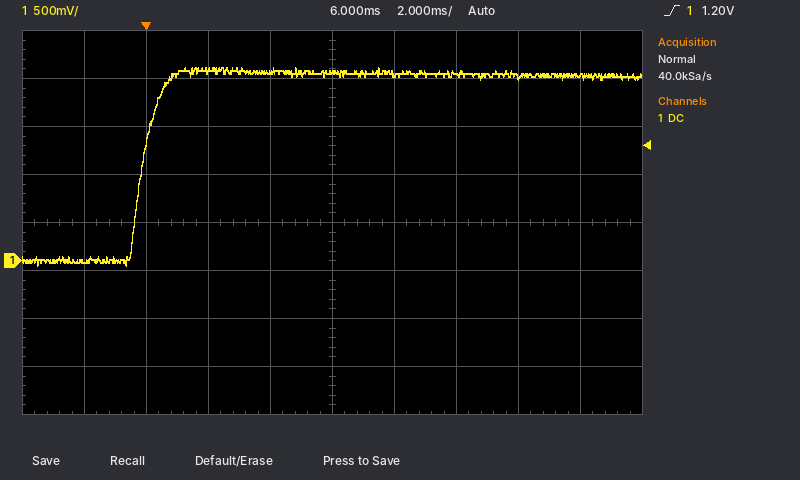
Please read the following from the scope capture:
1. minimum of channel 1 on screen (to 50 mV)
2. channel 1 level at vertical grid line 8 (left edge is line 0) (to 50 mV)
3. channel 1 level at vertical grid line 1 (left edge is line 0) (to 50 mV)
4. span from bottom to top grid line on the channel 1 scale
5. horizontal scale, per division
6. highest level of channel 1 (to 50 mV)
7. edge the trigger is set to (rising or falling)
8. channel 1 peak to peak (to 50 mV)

-50 mV
1.90 V
0 mV
4 V
2 ms
2.00 V
rising
2.05 V
